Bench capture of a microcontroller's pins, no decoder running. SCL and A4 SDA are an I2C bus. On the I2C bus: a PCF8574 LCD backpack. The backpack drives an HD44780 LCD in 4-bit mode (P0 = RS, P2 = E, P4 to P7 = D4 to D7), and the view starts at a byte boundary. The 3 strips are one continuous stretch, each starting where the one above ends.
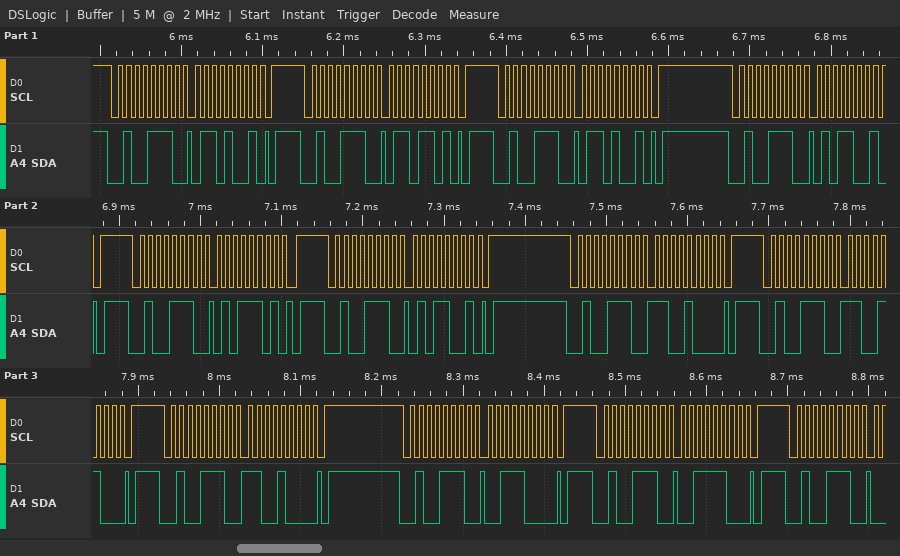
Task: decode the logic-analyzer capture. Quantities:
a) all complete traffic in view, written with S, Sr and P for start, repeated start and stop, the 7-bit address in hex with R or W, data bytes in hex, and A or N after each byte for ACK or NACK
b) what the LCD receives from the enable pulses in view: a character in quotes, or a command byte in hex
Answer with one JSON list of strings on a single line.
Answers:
["S 27W A 69 A P S 27W A 6D A P S 27W A 69 A P S 27W A 59 A P S 27W A 5D A P S 27W A 59 A P S 27W A C8 A P S 27W A CC A P S 27W A C8 A P S 27W A 38 A P S 27W A 3C A P S 27W A", "'e'"]
